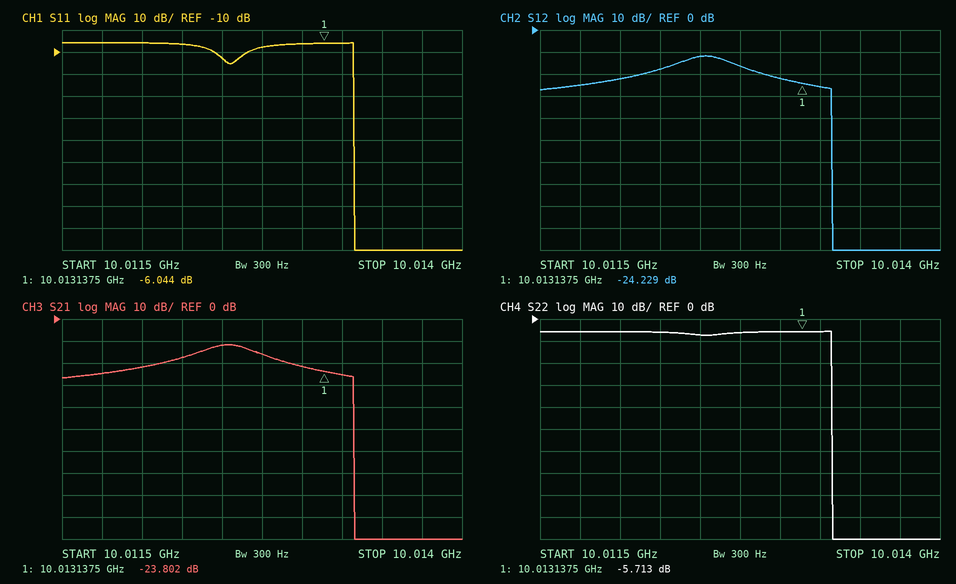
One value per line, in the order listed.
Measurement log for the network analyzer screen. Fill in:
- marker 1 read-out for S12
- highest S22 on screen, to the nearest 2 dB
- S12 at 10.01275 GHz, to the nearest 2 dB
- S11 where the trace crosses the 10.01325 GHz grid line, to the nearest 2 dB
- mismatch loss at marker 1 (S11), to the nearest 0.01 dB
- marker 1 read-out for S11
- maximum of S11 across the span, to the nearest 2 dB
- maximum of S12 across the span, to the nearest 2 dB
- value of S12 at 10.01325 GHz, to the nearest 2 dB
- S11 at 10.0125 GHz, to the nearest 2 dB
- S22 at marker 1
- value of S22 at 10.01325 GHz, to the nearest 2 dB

-24.229 dB
-6 dB
-16 dB
-6 dB
1.24 dB
-6.044 dB
-6 dB
-12 dB
-26 dB
-12 dB
-5.713 dB
-6 dB
